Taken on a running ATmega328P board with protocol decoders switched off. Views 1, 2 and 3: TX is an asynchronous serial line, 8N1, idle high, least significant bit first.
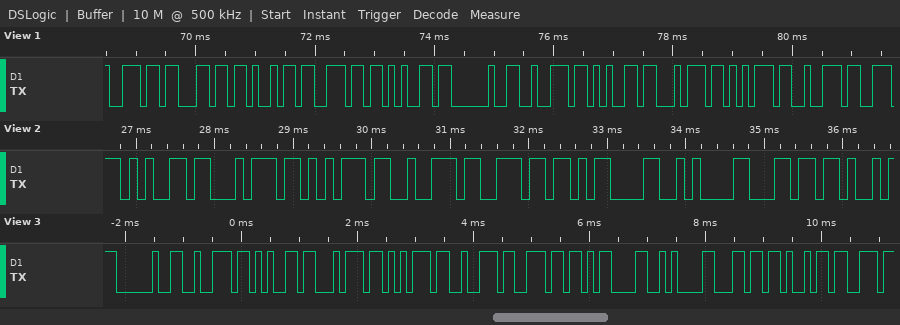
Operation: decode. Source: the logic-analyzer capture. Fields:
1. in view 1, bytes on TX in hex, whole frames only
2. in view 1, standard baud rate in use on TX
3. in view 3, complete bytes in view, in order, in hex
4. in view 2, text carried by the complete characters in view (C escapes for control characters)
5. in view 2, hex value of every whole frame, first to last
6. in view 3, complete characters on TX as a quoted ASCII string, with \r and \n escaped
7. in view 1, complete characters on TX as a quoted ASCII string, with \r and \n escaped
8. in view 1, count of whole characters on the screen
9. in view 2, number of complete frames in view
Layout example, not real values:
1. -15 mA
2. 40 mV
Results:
1. 0x6E 0x6C 0x69 0x6E 0x65 0x20 0x72 0x65 0x74 0x75 0x72
2. 9600 baud
3. 20 72 65 74 75 72 6E 0D 0A 6C 69
4. "eturn\r\nl"
5. 0x65 0x74 0x75 0x72 0x6E 0x0D 0x0A 0x6C
6. " return\r\nli"
7. "nline retur"
8. 11
9. 8
